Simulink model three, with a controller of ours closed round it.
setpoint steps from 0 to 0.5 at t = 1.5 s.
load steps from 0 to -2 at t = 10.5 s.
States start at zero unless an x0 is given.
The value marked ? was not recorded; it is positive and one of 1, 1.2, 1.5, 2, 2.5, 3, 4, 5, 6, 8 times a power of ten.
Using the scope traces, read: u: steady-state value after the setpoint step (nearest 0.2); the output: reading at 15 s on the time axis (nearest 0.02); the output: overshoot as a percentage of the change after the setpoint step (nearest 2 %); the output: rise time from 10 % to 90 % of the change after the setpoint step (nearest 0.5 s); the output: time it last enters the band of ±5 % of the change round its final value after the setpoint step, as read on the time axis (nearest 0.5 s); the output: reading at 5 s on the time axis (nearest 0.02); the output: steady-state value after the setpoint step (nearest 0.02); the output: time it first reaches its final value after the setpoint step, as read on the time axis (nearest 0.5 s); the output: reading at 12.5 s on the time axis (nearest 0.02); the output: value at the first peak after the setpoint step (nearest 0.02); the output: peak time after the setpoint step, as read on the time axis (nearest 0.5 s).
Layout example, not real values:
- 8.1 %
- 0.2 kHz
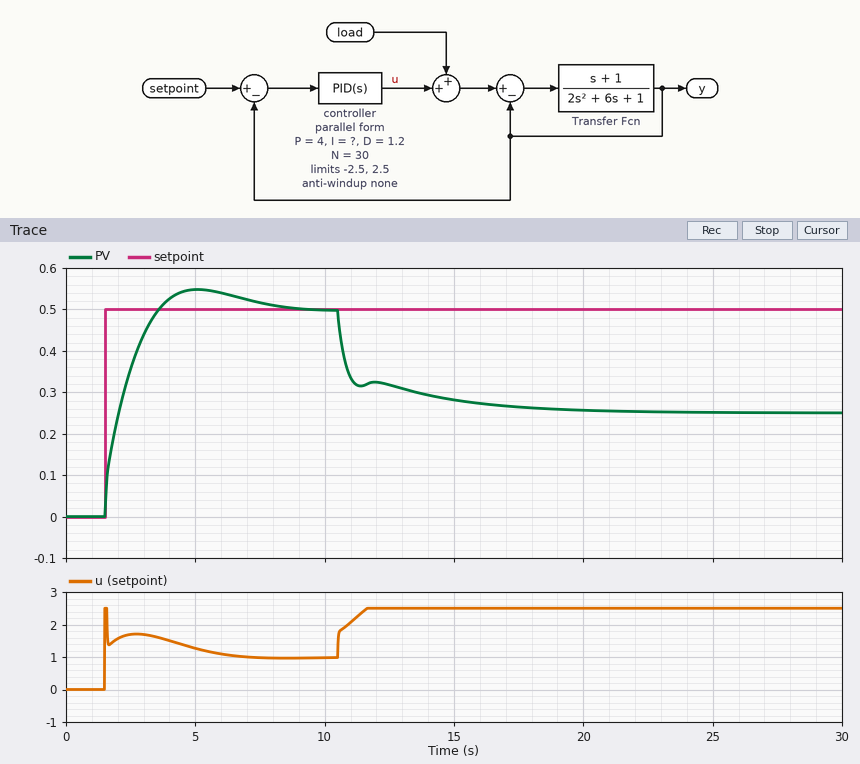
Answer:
- 1.0
- 0.28
- 10 %
- 1.5 s
- 7.0 s
- 0.54
- 0.50
- 3.5 s
- 0.32
- 0.54
- 5.0 s
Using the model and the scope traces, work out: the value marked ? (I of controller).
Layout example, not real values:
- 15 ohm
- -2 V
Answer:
- 5
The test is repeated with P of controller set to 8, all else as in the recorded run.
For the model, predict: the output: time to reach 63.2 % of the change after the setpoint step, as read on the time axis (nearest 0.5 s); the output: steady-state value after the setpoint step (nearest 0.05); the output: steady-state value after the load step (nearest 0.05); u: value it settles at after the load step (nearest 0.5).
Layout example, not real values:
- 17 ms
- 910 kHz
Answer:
- 2.0 s
- 0.50
- 0.25
- 2.5
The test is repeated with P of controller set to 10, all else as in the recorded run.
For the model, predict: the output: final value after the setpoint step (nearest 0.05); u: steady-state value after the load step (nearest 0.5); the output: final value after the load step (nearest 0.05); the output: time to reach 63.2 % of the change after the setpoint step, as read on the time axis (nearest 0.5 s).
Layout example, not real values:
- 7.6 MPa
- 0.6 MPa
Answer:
- 0.50
- 2.5
- 0.25
- 2.0 s
